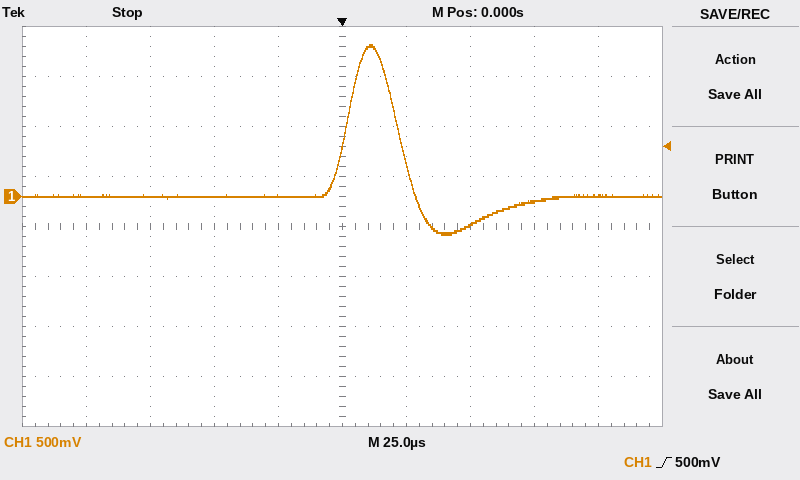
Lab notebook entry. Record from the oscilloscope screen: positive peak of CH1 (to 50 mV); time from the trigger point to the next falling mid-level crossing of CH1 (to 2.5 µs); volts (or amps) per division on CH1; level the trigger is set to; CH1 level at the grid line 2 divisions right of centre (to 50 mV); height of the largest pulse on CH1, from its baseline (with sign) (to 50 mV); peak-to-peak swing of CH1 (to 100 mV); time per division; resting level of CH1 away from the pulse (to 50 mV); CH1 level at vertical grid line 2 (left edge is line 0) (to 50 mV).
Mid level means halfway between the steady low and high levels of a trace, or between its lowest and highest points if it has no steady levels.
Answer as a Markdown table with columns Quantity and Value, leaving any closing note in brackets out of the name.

| Quantity | Value |
|---|---|
| positive peak of CH1 | 1.50 V |
| time from the trigger point to the next falling mid-level crossing of CH1 | 22.5 µs |
| volts (or amps) per division on CH1 | 500 mV |
| level the trigger is set to | 500 mV |
| CH1 level at the grid line 2 divisions right of centre | -300 mV |
| height of the largest pulse on CH1, from its baseline (with sign) | +1.50 V |
| peak-to-peak swing of CH1 | 1.90 V |
| time per division | 25 µs |
| resting level of CH1 away from the pulse | 0 mV |
| CH1 level at vertical grid line 2 (left edge is line 0) | 0 mV |
